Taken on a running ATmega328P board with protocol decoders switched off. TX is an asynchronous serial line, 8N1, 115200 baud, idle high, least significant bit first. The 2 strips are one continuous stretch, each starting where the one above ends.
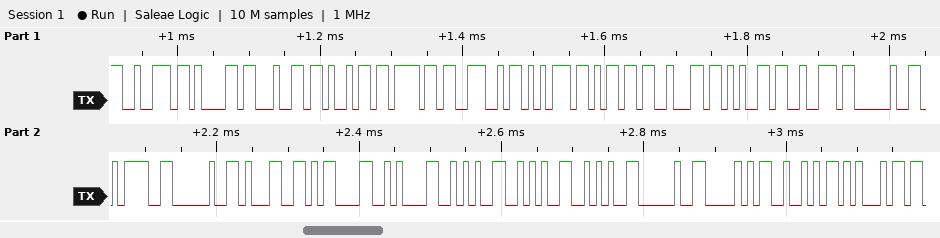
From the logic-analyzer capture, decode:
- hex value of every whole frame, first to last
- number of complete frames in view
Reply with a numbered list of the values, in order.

1. 72 61 64 69 6F 4E 75 6D 62 65 72 20 3D 20 31 0D 0A 2A 2A 2A 20 50 52 45
2. 24
